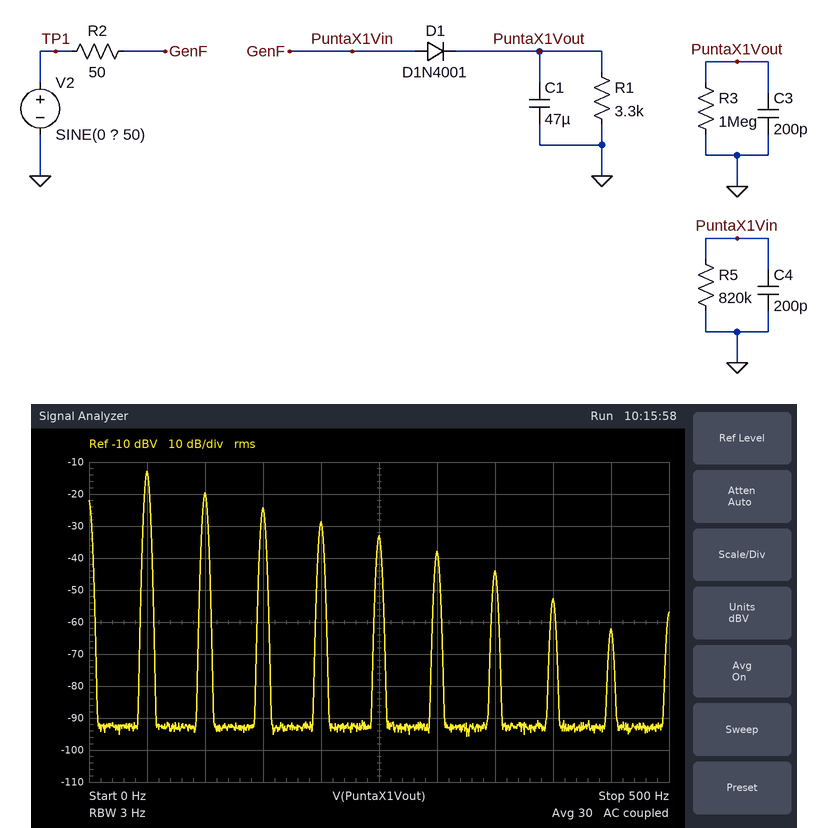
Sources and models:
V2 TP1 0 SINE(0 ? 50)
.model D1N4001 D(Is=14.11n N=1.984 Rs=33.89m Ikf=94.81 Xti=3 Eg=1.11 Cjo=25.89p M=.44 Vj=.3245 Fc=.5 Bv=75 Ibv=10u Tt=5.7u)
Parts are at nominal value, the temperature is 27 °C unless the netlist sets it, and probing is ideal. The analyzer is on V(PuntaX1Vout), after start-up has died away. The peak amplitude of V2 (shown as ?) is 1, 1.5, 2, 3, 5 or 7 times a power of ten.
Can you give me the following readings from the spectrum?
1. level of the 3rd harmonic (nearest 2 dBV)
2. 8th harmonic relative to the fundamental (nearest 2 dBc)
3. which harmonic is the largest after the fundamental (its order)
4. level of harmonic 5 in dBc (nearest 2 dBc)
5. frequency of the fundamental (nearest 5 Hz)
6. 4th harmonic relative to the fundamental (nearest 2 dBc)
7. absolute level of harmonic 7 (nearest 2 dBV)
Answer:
-24 dBV
-40 dBc
2
-20 dBc
50 Hz
-16 dBc
-44 dBV
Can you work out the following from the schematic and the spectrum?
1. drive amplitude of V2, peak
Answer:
10 V
